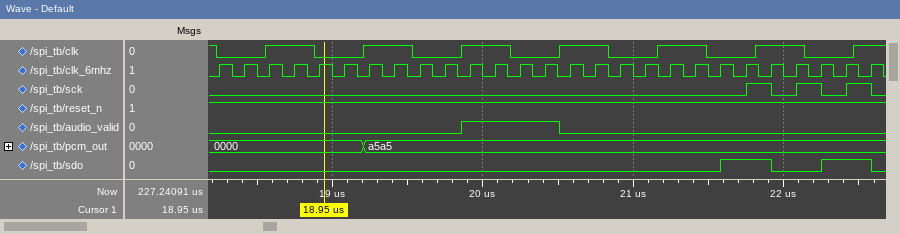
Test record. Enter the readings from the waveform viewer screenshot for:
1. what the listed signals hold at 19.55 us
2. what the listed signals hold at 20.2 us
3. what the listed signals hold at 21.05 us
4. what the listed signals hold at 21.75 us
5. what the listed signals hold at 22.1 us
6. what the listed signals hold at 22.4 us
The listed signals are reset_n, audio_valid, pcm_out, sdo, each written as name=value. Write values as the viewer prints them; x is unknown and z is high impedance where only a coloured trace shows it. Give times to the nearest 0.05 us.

reset_n=1, audio_valid=0, pcm_out=a5a5, sdo=0
reset_n=1, audio_valid=1, pcm_out=a5a5, sdo=0
reset_n=1, audio_valid=0, pcm_out=a5a5, sdo=0
reset_n=1, audio_valid=0, pcm_out=a5a5, sdo=1
reset_n=1, audio_valid=0, pcm_out=a5a5, sdo=0
reset_n=1, audio_valid=0, pcm_out=a5a5, sdo=1
